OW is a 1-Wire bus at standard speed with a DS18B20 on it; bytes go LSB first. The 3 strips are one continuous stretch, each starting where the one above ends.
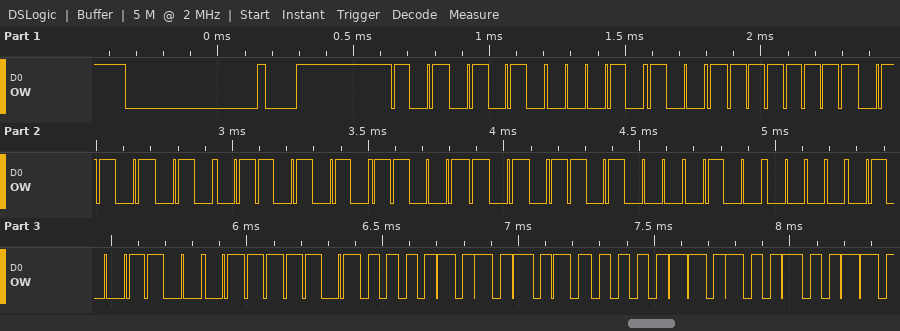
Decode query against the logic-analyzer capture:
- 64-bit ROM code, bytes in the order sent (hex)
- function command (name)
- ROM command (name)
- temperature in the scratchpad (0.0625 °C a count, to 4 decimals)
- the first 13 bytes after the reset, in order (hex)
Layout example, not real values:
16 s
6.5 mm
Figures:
28 FF 56 56 B3 16 02 32
Read Scratchpad
Match ROM
85.0000 °C
55 28 FF 56 56 B3 16 02 32 BE 50 05 4B
